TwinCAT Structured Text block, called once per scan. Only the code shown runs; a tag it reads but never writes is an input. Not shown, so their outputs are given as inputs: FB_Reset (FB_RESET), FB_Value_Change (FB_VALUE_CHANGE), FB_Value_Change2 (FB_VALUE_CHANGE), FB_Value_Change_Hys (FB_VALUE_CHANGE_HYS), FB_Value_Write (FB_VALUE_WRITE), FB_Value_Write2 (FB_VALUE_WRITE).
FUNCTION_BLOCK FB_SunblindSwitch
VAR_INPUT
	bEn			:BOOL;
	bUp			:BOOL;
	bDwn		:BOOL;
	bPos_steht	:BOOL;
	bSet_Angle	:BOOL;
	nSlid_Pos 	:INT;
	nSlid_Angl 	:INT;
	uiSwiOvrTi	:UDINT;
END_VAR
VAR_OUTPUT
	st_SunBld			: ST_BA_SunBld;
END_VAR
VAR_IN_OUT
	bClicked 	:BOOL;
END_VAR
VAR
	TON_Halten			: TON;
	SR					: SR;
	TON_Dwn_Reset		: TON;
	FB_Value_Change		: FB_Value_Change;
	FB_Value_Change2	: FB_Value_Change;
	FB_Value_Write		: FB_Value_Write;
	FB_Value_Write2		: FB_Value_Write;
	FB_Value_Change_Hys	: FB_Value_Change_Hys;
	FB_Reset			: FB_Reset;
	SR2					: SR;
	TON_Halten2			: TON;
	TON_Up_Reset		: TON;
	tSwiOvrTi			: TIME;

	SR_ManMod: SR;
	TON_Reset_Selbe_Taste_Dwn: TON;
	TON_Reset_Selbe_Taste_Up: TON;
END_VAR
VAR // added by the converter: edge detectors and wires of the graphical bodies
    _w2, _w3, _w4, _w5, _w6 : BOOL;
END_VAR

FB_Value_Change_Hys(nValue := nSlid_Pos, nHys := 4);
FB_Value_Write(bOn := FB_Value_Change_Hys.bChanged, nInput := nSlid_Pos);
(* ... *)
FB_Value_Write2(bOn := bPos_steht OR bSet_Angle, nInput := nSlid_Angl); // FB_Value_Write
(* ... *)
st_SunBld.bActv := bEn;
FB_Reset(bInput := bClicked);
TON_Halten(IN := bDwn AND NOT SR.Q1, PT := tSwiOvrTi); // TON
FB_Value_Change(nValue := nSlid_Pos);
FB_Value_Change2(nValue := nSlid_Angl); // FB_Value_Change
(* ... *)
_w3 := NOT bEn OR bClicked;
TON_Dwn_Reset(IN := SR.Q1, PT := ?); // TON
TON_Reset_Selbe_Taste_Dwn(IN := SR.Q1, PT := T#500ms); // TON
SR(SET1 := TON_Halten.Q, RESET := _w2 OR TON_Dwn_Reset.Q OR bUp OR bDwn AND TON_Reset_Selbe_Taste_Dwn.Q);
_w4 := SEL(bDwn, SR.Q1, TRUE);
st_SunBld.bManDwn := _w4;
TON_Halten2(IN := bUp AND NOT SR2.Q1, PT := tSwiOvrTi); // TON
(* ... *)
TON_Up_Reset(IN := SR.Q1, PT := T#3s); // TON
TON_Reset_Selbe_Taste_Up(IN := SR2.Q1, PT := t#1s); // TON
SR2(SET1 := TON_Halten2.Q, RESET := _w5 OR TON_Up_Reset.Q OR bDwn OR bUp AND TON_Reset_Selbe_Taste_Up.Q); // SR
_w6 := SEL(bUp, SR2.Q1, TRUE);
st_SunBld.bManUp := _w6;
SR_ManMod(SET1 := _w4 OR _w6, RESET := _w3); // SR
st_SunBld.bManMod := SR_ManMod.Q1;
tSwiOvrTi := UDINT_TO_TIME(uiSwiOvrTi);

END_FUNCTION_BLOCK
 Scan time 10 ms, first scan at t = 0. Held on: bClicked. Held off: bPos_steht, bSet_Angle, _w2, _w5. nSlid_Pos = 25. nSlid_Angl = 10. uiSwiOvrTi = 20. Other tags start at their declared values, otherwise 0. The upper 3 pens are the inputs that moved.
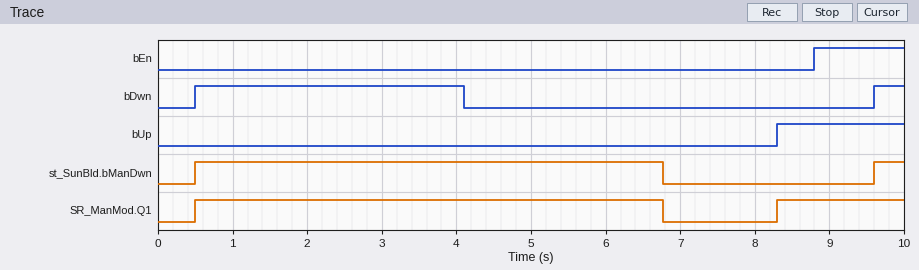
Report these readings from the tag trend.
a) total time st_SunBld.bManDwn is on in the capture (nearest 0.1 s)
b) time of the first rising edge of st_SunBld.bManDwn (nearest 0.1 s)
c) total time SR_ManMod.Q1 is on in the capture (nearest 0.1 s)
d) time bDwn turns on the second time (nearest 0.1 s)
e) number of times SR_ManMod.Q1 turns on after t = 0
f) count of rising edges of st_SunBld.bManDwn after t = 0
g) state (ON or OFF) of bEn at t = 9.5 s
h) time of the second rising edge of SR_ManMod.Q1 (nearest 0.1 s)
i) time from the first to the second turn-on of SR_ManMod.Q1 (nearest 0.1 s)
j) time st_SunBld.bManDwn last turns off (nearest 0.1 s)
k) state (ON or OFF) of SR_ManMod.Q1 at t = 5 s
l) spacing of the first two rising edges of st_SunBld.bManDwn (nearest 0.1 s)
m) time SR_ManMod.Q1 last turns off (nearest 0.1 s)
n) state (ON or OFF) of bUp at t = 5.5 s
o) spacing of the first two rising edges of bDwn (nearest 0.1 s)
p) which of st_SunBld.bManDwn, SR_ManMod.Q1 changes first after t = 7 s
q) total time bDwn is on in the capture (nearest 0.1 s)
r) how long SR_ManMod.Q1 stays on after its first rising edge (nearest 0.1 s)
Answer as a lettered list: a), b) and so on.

a) 6.7 s
b) 0.5 s
c) 8.0 s
d) 9.6 s
e) 2
f) 2
g) ON
h) 8.3 s
i) 7.8 s
j) 6.8 s
k) ON
l) 9.1 s
m) 6.8 s
n) OFF
o) 9.1 s
p) SR_ManMod.Q1
q) 4.0 s
r) 6.3 s
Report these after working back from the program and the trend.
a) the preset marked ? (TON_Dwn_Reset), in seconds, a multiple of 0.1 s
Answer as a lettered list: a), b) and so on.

a) 3.0 s
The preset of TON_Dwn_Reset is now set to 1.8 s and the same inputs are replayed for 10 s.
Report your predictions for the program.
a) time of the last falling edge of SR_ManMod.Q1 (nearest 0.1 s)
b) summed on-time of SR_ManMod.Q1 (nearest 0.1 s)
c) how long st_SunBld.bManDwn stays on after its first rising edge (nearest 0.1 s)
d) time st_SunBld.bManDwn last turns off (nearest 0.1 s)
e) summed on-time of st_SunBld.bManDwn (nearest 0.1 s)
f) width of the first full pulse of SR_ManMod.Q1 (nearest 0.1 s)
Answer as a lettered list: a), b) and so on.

a) 5.6 s
b) 6.8 s
c) 5.1 s
d) 5.6 s
e) 5.5 s
f) 5.1 s
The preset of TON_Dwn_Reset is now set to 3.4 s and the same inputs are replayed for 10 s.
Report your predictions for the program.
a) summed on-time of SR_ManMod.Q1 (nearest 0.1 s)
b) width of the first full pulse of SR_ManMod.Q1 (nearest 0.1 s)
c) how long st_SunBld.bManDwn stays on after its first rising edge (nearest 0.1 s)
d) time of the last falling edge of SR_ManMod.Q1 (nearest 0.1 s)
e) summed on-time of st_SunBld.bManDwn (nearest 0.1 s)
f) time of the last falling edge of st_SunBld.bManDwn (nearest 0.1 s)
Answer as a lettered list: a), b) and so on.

a) 8.4 s
b) 6.7 s
c) 6.7 s
d) 7.2 s
e) 7.1 s
f) 7.2 s
